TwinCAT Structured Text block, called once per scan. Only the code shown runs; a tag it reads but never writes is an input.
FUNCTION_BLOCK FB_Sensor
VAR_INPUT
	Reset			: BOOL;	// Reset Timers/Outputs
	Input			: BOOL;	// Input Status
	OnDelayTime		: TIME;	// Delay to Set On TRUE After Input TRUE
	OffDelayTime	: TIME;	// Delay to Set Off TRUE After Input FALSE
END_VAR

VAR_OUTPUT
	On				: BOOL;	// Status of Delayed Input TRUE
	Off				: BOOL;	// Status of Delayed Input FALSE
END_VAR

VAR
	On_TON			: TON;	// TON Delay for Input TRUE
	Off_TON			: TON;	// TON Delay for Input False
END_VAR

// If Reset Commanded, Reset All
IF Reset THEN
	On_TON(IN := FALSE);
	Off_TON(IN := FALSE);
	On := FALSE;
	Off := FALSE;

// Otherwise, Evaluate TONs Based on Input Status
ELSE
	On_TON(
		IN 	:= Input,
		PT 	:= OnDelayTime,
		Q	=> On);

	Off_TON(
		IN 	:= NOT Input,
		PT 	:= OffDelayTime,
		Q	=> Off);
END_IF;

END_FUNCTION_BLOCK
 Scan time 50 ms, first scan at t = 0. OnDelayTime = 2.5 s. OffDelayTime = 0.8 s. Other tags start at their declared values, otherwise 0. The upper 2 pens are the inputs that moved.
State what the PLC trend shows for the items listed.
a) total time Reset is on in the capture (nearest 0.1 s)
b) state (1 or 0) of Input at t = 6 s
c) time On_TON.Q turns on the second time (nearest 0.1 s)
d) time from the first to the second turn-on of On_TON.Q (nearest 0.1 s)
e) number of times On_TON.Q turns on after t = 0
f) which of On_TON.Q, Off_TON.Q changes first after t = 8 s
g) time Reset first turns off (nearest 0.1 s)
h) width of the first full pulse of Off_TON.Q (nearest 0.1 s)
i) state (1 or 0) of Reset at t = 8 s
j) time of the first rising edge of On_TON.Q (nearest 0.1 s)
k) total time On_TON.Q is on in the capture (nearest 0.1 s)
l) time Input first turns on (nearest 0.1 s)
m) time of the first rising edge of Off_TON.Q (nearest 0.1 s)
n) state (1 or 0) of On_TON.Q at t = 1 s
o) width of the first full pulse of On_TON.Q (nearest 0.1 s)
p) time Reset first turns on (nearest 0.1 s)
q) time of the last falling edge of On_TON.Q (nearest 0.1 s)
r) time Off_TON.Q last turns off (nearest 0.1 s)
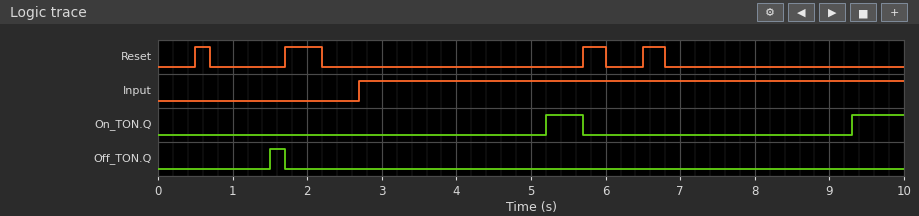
1.3 s
1
9.3 s
4.1 s
2
On_TON.Q
0.7 s
0.2 s
0
5.2 s
1.2 s
2.7 s
1.5 s
0
0.5 s
0.5 s
5.7 s
1.7 s
